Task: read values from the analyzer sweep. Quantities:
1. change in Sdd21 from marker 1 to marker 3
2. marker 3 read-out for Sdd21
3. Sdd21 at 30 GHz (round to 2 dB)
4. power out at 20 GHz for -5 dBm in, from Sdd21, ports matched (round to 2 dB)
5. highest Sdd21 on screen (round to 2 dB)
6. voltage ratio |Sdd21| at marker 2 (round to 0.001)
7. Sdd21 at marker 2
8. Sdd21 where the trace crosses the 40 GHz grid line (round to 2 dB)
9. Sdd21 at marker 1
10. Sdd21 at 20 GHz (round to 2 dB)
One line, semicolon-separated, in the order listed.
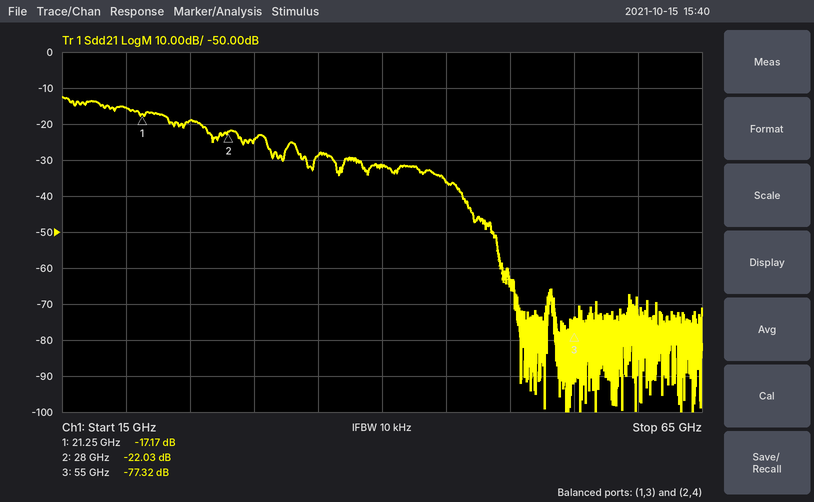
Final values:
-60.15 dB; -77.32 dB; -24 dB; -20 dBm; -12 dB; 0.079; -22.03 dB; -32 dB; -17.17 dB; -16 dB
